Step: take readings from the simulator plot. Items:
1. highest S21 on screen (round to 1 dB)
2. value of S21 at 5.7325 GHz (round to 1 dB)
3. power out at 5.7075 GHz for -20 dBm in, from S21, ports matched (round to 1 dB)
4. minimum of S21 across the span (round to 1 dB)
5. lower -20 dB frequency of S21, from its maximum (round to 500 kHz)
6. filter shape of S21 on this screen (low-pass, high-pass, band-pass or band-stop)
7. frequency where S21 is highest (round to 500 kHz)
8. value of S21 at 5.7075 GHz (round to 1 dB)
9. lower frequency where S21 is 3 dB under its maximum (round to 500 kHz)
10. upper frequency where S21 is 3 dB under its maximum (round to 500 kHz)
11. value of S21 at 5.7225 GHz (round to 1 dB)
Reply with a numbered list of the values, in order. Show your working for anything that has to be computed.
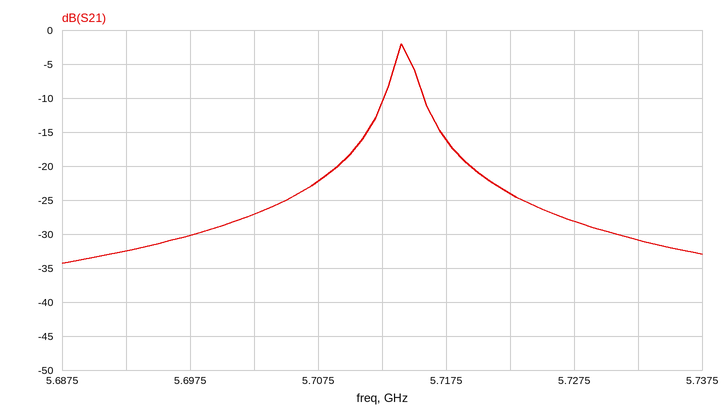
1. -2 dB
2. -31 dB
3. -20 dBm + (-22 dB) = -42 dBm
4. -34 dB
5. 5.7075 GHz
6. band-pass
7. 5.7140 GHz
8. -22 dB
9. 5.7135 GHz
10. 5.7150 GHz
11. -24 dB
